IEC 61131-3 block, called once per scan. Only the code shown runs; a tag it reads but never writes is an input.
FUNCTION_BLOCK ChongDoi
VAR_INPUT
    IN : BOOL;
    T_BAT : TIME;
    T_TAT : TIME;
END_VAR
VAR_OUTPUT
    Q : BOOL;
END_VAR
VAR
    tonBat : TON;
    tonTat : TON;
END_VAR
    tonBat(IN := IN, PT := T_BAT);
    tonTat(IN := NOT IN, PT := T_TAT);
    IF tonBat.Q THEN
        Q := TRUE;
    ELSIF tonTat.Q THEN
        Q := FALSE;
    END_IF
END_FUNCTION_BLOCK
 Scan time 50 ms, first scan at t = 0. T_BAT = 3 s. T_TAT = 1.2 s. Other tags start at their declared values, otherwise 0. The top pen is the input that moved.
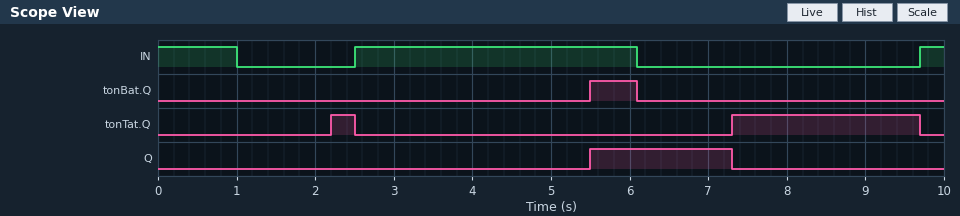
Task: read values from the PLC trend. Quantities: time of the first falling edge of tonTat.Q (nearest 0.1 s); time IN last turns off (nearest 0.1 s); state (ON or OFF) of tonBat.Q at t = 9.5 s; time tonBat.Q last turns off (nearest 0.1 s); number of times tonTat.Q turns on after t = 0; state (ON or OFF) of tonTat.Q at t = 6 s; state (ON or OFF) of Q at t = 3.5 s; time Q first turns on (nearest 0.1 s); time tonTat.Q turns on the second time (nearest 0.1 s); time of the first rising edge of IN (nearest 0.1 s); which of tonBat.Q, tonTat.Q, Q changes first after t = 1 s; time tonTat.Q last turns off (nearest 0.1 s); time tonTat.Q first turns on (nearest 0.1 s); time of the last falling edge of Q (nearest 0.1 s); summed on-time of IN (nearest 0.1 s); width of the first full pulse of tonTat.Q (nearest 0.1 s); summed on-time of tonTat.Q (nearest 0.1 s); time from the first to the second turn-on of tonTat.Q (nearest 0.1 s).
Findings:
2.5 s
6.1 s
OFF
6.1 s
2
OFF
OFF
5.5 s
7.3 s
2.5 s
tonTat.Q
9.7 s
2.2 s
7.3 s
4.9 s
0.3 s
2.7 s
5.1 s
